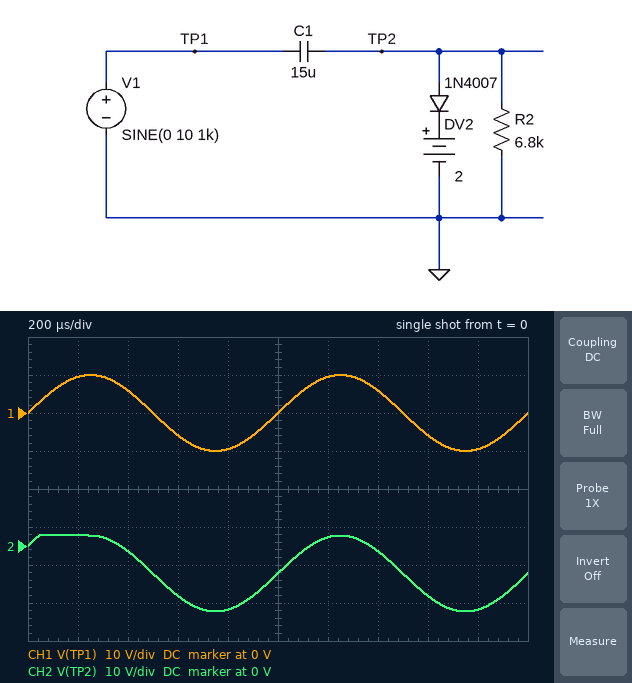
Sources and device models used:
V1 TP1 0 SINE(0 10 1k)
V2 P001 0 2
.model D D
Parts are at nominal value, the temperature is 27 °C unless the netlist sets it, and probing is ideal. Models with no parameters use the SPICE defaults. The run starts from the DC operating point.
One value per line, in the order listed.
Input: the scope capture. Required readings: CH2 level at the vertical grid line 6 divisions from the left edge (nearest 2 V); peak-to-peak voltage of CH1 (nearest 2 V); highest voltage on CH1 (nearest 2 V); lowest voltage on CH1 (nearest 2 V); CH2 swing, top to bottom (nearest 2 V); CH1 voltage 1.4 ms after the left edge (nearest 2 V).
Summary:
2 V
20 V
10 V
-10 V
20 V
6 V
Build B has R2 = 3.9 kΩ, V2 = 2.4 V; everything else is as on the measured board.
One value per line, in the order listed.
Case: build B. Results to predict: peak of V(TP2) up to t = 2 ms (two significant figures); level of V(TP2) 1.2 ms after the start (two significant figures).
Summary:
3.2 V
2.8 V
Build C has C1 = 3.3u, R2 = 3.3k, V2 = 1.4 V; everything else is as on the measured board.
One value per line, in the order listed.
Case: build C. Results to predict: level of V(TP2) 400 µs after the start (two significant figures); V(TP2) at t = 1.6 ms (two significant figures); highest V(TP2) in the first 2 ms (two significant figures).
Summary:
-2.0 V
-14 V
2.2 V
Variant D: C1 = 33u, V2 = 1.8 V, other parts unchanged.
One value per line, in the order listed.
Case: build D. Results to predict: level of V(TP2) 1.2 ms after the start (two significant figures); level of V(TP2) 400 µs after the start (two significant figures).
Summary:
2.1 V
-1.6 V
